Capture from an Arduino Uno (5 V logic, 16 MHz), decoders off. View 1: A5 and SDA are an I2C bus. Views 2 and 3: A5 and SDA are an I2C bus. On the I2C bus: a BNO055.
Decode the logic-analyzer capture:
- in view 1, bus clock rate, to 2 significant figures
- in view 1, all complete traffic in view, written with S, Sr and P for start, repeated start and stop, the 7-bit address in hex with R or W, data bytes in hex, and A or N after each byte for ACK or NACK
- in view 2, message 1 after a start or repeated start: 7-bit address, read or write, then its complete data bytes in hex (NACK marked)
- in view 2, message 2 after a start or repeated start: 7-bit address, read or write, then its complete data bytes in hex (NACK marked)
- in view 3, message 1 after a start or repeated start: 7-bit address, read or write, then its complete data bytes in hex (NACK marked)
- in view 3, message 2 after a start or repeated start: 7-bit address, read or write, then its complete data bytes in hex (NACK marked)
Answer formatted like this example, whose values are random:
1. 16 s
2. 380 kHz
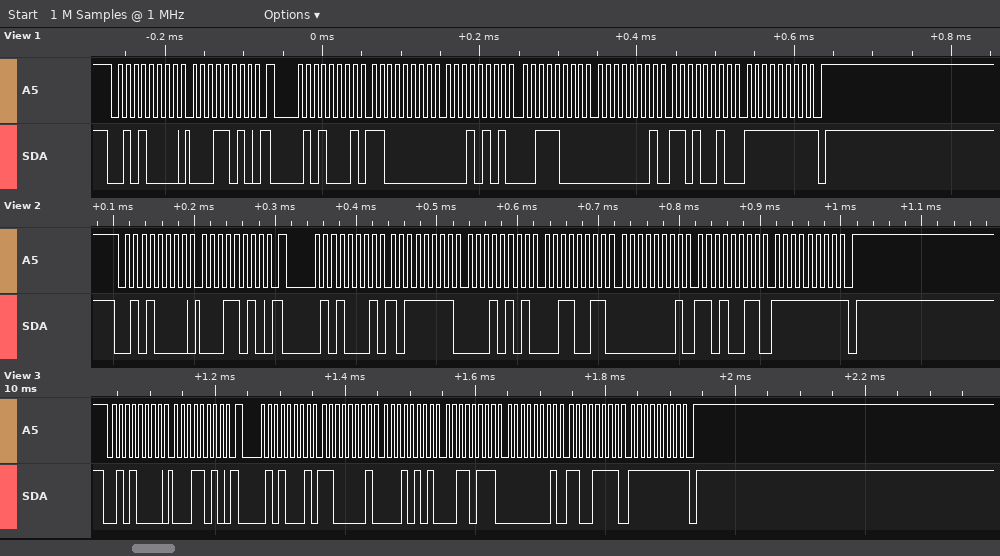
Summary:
1. 100 kHz
2. S 28W A 1A A Sr 28R A C0 A 15 A 38 A 01 A D2 A FF N P
3. 0x28 write: 1A
4. 0x28 read: BF 15 33 01 D3 FF NACK
5. 0x28 write: 1A
6. 0x28 read: C1 15 37 01 CF FF NACK
